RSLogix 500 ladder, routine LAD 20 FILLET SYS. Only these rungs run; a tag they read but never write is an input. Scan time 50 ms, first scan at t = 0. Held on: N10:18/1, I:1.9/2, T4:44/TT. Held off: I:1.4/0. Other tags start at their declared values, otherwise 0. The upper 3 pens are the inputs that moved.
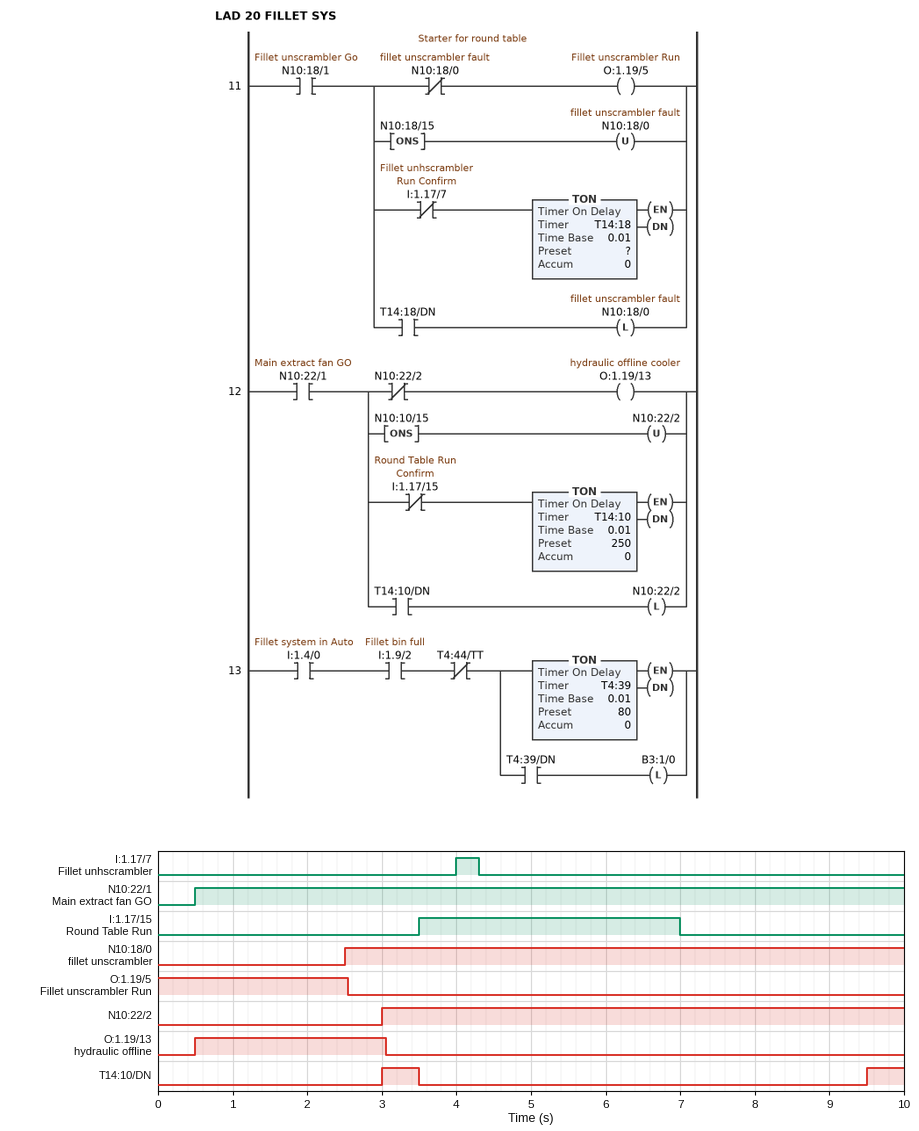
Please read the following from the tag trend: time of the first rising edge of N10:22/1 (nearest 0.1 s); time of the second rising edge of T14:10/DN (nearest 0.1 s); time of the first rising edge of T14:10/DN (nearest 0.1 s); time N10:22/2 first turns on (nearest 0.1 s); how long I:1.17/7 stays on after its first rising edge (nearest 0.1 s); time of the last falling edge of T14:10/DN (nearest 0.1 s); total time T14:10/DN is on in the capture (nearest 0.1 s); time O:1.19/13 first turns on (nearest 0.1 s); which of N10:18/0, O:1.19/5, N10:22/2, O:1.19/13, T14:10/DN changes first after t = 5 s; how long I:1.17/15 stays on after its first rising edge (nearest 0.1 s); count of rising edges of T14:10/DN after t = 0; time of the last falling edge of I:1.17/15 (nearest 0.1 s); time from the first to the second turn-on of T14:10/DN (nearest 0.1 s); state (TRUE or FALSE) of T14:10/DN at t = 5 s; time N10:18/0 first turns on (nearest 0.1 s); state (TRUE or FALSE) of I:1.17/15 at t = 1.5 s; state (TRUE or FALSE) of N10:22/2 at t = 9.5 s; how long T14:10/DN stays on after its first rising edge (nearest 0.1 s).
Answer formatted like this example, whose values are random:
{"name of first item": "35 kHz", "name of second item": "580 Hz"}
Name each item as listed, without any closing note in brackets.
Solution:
{"time of the first rising edge of N10:22/1": "0.5 s", "time of the second rising edge of T14:10/DN": "9.5 s", "time of the first rising edge of T14:10/DN": "3.0 s", "time N10:22/2 first turns on": "3.0 s", "how long I:1.17/7 stays on after its first rising edge": "0.3 s", "time of the last falling edge of T14:10/DN": "3.5 s", "total time T14:10/DN is on in the capture": "1.0 s", "time O:1.19/13 first turns on": "0.5 s", "which of N10:18/0, O:1.19/5, N10:22/2, O:1.19/13, T14:10/DN changes first after t = 5 s": "T14:10/DN", "how long I:1.17/15 stays on after its first rising edge": "3.5 s", "count of rising edges of T14:10/DN after t = 0": "2", "time of the last falling edge of I:1.17/15": "7.0 s", "time from the first to the second turn-on of T14:10/DN": "6.5 s", "state (TRUE or FALSE) of T14:10/DN at t = 5 s": "FALSE", "time N10:18/0 first turns on": "2.5 s", "state (TRUE or FALSE) of I:1.17/15 at t = 1.5 s": "FALSE", "state (TRUE or FALSE) of N10:22/2 at t = 9.5 s": "TRUE", "how long T14:10/DN stays on after its first rising edge": "0.5 s"}
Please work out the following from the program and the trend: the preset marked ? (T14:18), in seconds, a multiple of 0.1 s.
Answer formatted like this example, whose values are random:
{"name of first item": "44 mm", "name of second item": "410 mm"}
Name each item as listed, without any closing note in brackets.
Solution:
{"the preset marked ? (T14:18), in seconds, a multiple of 0.1 s": "2.5 s"}
